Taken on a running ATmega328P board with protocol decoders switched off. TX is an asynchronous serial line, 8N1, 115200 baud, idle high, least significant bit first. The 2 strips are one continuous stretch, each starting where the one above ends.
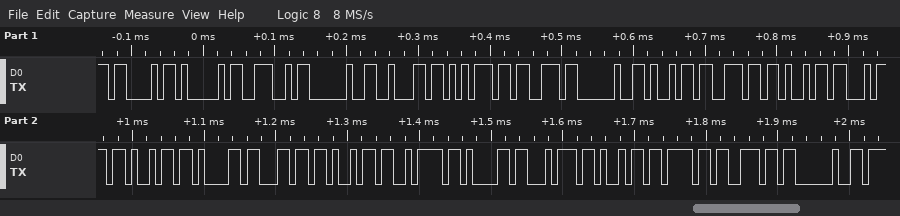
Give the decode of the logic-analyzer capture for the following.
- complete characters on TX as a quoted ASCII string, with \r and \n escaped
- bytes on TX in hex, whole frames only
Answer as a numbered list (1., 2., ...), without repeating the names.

1. "CAN bus initialization "
2. 43 41 4E 20 62 75 73 20 69 6E 69 74 69 61 6C 69 7A 61 74 69 6F 6E 20
